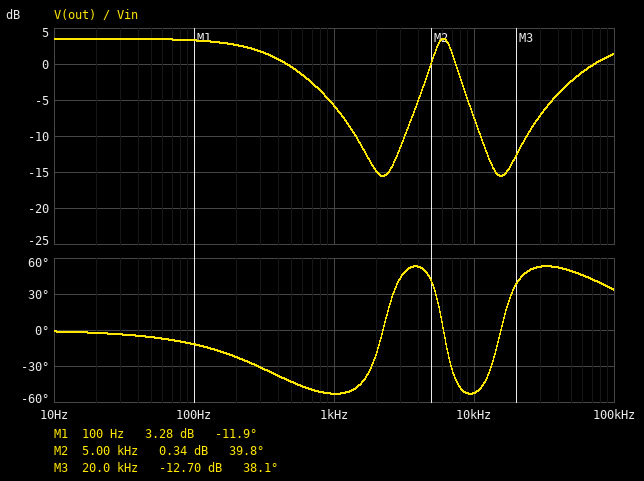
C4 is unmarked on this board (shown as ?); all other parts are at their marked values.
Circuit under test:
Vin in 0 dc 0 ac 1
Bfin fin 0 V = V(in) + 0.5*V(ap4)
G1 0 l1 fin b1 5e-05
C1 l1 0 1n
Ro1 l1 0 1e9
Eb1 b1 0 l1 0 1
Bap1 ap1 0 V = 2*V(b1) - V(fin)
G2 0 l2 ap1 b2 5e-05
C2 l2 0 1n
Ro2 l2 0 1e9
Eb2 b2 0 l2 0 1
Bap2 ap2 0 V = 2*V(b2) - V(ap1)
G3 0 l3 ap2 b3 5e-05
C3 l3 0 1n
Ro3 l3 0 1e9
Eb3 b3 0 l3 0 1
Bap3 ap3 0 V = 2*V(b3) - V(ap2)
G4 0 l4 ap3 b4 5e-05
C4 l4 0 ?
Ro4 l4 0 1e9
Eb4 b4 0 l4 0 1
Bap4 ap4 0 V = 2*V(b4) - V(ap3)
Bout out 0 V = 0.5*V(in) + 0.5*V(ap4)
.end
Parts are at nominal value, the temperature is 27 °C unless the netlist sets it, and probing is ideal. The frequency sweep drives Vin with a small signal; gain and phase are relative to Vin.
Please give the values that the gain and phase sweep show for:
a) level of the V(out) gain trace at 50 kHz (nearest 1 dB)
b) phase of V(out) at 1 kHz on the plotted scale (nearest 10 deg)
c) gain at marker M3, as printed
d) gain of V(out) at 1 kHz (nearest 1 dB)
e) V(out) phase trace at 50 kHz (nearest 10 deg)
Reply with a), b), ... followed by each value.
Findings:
a) -2 dB
b) -50 deg
c) -12.70 dB
d) -6 dB
e) 50 deg
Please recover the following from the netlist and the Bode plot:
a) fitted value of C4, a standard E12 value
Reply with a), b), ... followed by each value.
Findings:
a) 3.3 nF
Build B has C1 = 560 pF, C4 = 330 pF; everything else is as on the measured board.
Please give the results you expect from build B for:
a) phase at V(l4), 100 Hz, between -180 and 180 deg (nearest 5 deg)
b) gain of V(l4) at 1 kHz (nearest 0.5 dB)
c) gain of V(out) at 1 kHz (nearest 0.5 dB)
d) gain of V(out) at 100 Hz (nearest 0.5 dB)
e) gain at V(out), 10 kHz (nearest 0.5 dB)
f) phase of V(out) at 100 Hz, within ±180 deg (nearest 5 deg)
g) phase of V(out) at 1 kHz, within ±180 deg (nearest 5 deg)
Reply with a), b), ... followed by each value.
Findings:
a) -10 deg
b) 3.0 dB
c) 0 dB
d) 3.5 dB
e) 0.5 dB
f) -5 deg
g) -40 deg
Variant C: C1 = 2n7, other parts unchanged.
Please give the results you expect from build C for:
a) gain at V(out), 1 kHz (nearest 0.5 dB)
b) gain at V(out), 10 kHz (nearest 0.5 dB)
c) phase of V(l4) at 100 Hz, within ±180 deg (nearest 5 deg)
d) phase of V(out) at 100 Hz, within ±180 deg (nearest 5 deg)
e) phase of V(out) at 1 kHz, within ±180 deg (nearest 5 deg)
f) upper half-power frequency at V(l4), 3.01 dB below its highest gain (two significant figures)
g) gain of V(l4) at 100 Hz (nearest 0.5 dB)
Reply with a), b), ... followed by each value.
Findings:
a) -8.5 dB
b) -13.0 dB
c) -20 deg
d) -15 deg
e) -50 deg
f) 350 Hz
g) 5.5 dB
